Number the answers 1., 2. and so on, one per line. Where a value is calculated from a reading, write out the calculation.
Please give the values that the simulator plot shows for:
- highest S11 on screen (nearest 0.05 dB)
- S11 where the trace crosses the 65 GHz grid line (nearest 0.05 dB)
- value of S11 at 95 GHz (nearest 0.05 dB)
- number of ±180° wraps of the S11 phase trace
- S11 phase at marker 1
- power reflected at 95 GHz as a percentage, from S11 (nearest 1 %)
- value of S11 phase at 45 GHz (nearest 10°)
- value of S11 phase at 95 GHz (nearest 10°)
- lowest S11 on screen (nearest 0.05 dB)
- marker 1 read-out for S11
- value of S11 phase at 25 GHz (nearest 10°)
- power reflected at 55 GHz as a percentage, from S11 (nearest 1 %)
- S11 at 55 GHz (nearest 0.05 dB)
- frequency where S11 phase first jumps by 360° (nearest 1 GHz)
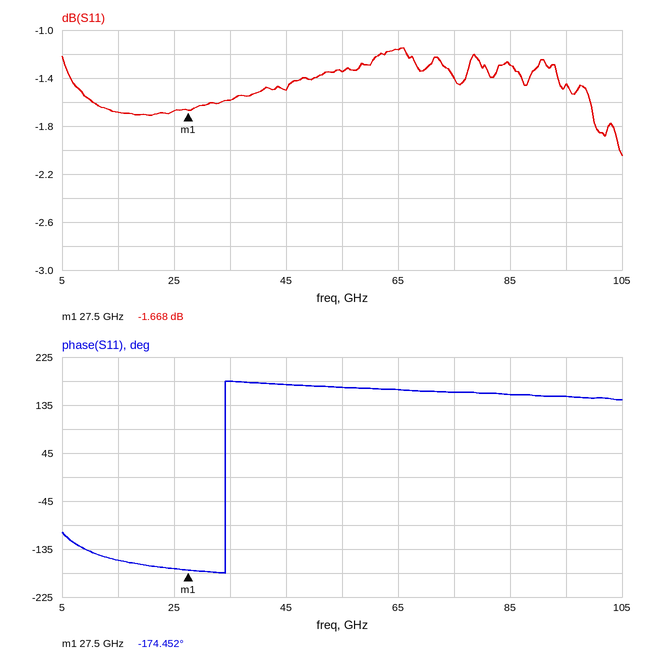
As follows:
1. -1.15 dB
2. -1.15 dB
3. -1.45 dB
4. 1
5. -174.452°
6. 10^(-1.45/10) ≈ 72 %
7. 170°
8. 150°
9. -2.05 dB
10. -1.668 dB
11. -170°
12. 10^(-1.35/10) ≈ 73 %
13. -1.35 dB
14. 34 GHz
